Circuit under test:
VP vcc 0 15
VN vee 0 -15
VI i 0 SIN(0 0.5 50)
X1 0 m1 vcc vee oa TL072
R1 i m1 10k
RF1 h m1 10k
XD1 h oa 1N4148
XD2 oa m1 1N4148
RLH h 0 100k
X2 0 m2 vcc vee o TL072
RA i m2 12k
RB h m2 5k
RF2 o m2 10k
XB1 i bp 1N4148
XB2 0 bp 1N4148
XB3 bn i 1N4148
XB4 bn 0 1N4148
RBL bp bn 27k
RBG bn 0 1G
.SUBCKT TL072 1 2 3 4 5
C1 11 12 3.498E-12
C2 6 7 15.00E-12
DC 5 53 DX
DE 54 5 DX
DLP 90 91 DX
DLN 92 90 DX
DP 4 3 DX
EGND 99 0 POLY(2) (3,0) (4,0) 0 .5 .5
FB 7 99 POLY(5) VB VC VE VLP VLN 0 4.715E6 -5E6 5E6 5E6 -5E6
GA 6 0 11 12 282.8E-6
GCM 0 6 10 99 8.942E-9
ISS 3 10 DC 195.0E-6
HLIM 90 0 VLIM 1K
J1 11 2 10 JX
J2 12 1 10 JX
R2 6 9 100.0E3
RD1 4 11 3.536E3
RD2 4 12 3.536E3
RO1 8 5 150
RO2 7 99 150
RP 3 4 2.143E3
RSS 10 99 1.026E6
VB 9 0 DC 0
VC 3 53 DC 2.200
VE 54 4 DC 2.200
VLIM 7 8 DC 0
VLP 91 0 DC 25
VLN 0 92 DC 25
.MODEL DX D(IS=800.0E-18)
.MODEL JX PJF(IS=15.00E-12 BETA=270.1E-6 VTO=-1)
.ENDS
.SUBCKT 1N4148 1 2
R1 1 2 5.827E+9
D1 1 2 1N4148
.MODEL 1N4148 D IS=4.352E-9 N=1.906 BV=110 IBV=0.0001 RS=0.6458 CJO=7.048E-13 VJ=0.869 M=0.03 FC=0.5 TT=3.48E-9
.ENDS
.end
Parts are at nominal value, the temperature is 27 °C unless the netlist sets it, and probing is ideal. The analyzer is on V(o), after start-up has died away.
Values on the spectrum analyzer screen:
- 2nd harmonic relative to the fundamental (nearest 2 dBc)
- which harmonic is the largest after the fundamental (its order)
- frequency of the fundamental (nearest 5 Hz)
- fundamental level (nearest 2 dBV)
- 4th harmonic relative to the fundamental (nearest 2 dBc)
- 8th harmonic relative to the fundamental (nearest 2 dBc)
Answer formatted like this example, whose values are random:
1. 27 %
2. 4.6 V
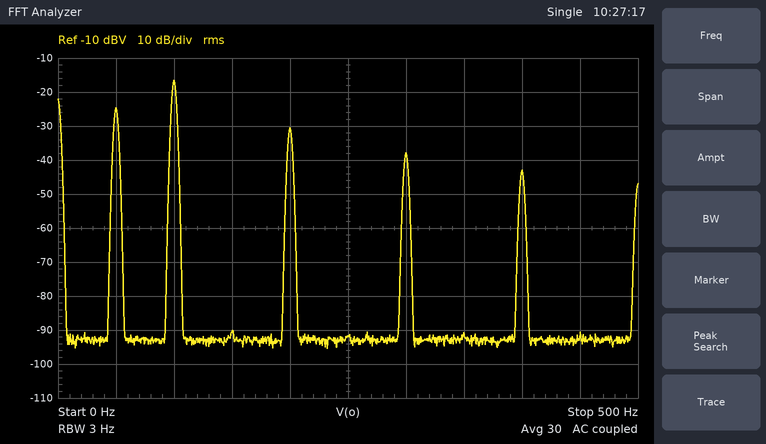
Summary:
1. 8 dBc
2. 2
3. 50 Hz
4. -24 dBV
5. -6 dBc
6. -18 dBc
